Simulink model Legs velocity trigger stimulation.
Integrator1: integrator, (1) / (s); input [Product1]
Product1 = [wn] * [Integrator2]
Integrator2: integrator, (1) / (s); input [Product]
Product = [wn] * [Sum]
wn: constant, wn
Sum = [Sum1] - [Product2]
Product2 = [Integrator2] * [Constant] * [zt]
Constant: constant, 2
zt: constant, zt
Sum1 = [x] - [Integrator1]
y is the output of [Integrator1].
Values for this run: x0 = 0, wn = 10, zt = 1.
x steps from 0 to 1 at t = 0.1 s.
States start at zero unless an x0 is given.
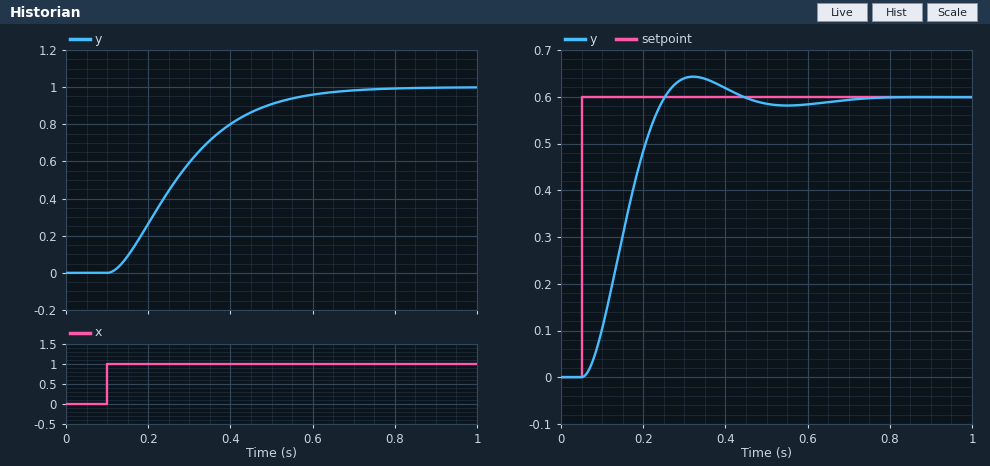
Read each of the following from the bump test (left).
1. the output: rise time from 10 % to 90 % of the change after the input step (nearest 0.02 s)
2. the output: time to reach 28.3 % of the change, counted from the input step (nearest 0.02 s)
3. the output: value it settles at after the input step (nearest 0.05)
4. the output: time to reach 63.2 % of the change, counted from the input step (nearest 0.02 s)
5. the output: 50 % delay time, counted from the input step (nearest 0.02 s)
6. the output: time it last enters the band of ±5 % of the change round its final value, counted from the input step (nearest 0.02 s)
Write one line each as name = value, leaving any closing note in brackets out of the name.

the output: rise time from 10 % to 90 % of the change after the input step = 0.34 s
the output: time to reach 28.3 % of the change, counted from the input step = 0.10 s
the output: value it settles at after the input step = 1.00
the output: time to reach 63.2 % of the change, counted from the input step = 0.22 s
the output: 50 % delay time, counted from the input step = 0.16 s
the output: time it last enters the band of ±5 % of the change round its final value, counted from the input step = 0.48 s
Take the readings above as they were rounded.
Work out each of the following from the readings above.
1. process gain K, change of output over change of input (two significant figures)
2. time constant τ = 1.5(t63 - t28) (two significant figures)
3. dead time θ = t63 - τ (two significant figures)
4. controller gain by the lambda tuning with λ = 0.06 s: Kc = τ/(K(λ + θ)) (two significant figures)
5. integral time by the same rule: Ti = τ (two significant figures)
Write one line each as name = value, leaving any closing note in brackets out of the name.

process gain K, change of output over change of input = 1.0
time constant τ = 1.5(t63 - t28) = 0.18 s
dead time θ = t63 - τ = 0.040 s
controller gain by the lambda tuning with λ = 0.06 s: Kc = τ/(K(λ + θ)) = 1.8
integral time by the same rule: Ti = τ = 0.18 s
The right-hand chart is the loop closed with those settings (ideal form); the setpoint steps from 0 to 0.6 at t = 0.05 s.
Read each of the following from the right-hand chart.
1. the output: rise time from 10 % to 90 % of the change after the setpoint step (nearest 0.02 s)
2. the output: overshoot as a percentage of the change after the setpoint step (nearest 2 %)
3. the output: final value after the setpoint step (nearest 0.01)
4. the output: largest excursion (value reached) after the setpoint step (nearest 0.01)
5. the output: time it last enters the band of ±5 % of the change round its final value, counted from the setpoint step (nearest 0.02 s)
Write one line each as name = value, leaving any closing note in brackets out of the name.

the output: rise time from 10 % to 90 % of the change after the setpoint step = 0.14 s
the output: overshoot as a percentage of the change after the setpoint step = 8 %
the output: final value after the setpoint step = 0.60
the output: largest excursion (value reached) after the setpoint step = 0.64
the output: time it last enters the band of ±5 % of the change round its final value, counted from the setpoint step = 0.32 s
